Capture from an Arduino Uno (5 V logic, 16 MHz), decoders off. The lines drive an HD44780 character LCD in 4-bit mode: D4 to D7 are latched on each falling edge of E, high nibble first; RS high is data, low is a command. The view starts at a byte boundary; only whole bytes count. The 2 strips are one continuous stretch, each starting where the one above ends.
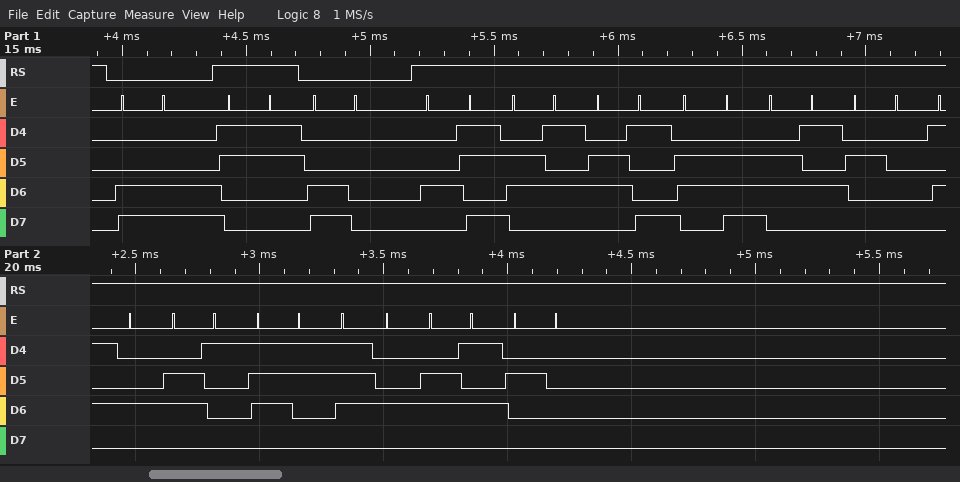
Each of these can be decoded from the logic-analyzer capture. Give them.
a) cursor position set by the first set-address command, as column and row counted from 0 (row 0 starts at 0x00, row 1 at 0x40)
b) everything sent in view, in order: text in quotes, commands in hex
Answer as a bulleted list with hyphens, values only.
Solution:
- column 12, row 1
- 0xCC "3" 0xC0 "Keine Taste "
